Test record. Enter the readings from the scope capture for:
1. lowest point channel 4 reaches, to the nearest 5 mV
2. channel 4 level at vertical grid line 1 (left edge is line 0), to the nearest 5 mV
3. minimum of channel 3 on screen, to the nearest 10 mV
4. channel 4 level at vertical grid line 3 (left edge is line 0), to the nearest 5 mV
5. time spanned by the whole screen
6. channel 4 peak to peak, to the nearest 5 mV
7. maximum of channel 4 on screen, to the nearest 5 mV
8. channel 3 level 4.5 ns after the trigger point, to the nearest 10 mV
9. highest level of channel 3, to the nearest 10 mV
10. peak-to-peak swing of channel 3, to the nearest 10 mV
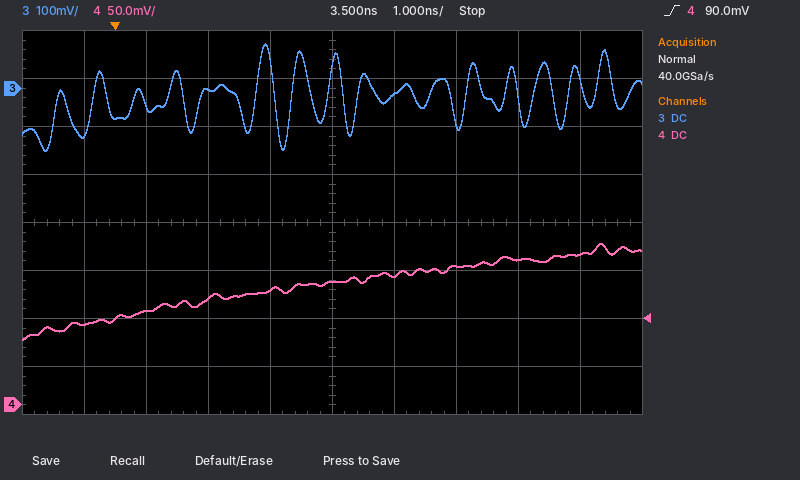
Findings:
70 mV
85 mV
-130 mV
110 mV
10 ns
100 mV
170 mV
-10 mV
90 mV
220 mV
